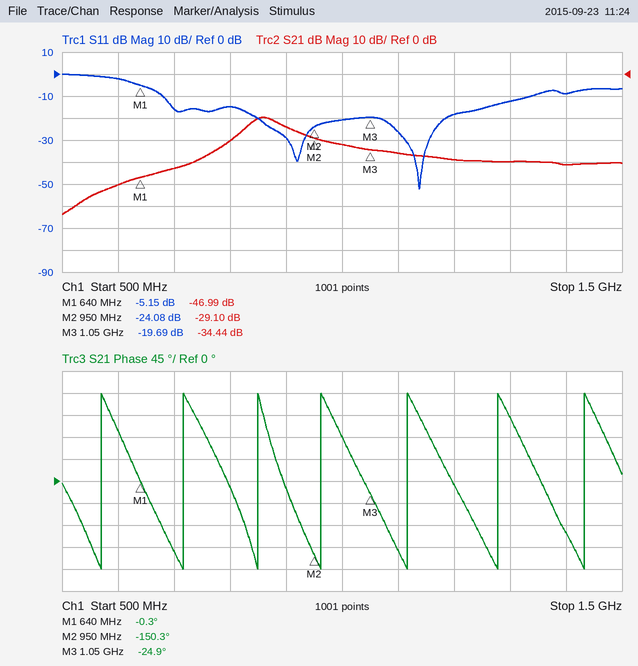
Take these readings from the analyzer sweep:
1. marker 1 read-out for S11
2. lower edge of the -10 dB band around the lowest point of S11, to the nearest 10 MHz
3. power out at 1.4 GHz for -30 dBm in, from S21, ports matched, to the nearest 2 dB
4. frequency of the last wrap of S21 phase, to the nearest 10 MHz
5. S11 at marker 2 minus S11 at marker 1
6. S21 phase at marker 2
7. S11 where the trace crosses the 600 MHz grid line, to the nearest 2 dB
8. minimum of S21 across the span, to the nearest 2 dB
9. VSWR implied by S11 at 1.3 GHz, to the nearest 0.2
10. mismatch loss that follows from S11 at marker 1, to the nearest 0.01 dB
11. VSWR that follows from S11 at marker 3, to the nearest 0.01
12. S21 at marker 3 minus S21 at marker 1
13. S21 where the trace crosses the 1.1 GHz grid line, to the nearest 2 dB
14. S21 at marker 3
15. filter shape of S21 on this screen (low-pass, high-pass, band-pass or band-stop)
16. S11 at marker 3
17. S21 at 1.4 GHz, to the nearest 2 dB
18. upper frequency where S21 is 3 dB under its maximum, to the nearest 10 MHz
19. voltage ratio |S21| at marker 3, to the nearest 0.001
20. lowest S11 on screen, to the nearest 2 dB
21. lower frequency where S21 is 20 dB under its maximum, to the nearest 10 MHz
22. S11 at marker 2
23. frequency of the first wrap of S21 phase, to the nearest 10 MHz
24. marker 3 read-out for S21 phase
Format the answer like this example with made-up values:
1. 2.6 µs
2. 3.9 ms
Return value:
1. -5.15 dB
2. 680 MHz
3. -72 dBm
4. 1.43 GHz
5. -18.93 dB
6. -150.3°
7. -2 dB
8. -64 dB
9. 1.6
10. 1.58 dB
11. 1.23
12. 12.55 dB
13. -36 dB
14. -34.44 dB
15. band-pass
16. -19.69 dB
17. -42 dB
18. 890 MHz
19. 0.019
20. -52 dB
21. 740 MHz
22. -24.08 dB
23. 570 MHz
24. -24.9°
